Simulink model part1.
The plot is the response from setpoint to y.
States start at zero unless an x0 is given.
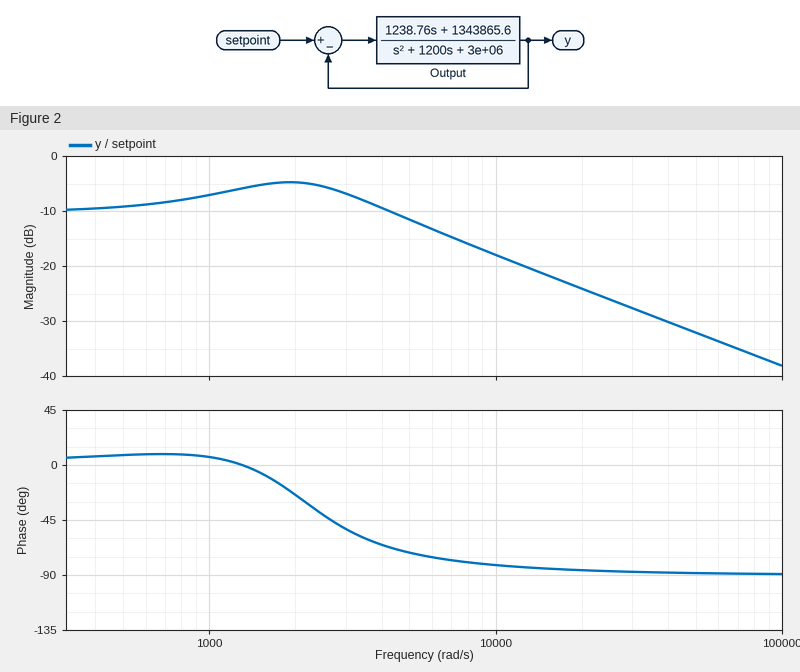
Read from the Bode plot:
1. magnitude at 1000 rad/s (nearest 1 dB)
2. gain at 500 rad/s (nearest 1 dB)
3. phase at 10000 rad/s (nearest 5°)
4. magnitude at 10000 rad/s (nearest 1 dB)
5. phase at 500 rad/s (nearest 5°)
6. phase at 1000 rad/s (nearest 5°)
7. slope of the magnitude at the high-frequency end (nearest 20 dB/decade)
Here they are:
-7 dB
-9 dB
-80°
-18 dB
10°
5°
-20 dB/decade
